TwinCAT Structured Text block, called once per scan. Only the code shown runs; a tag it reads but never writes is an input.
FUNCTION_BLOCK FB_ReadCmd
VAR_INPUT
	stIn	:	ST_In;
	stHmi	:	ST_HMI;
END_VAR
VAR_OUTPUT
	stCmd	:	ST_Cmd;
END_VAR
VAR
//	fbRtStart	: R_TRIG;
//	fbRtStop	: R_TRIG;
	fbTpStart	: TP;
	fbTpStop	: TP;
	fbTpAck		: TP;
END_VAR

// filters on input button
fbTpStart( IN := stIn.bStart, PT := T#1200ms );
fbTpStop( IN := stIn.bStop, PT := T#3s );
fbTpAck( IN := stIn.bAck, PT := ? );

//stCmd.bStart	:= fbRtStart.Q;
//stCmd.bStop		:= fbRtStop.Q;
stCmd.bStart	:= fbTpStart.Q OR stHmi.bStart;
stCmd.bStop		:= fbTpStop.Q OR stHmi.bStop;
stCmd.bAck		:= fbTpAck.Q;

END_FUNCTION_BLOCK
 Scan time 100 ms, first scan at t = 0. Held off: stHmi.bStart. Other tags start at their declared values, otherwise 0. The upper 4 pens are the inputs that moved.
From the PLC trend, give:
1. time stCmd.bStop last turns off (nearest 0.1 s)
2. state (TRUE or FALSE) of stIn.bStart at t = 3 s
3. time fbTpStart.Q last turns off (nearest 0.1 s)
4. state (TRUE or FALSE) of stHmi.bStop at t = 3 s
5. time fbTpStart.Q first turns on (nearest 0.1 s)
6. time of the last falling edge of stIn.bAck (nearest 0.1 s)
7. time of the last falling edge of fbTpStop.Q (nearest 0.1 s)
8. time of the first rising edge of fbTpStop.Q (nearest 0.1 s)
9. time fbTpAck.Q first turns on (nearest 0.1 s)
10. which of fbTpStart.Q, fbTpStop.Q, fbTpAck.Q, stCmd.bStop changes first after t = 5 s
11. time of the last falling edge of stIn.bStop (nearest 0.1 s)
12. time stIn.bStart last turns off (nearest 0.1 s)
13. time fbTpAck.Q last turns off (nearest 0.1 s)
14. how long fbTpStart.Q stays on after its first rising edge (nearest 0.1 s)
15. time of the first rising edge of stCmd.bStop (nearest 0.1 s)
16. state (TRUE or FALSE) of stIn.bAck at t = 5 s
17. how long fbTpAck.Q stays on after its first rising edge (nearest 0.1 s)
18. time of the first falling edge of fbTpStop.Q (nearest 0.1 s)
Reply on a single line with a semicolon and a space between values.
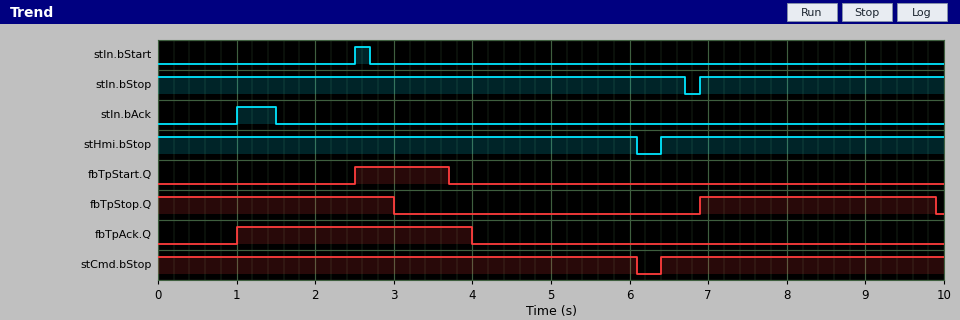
6.1 s; FALSE; 3.7 s; TRUE; 2.5 s; 1.5 s; 9.9 s; 6.9 s; 1.0 s; stCmd.bStop; 6.7 s; 2.7 s; 4.0 s; 1.2 s; 6.4 s; FALSE; 3.0 s; 3.0 s
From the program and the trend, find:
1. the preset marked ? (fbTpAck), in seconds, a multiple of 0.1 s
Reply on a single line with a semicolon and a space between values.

3.0 s
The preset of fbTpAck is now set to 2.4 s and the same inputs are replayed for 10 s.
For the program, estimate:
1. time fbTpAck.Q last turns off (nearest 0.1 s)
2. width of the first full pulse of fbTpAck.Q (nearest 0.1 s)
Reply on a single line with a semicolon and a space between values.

3.4 s; 2.4 s
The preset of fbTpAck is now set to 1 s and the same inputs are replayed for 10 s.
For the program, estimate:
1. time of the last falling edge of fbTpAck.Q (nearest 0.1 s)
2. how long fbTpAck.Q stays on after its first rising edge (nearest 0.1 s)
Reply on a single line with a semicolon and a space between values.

2.0 s; 1.0 s
